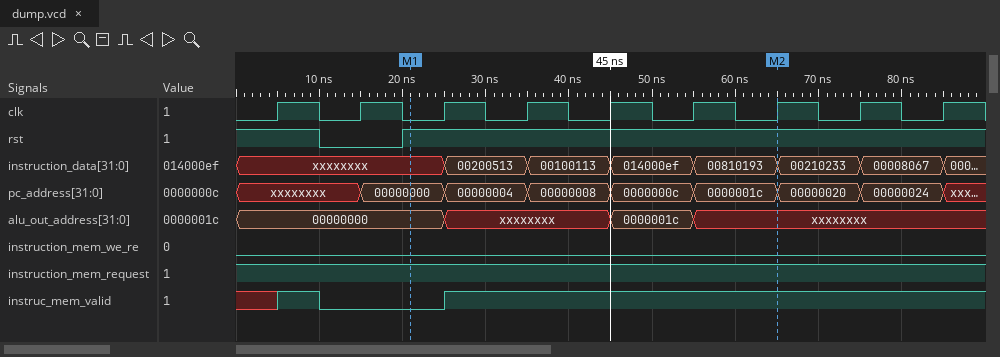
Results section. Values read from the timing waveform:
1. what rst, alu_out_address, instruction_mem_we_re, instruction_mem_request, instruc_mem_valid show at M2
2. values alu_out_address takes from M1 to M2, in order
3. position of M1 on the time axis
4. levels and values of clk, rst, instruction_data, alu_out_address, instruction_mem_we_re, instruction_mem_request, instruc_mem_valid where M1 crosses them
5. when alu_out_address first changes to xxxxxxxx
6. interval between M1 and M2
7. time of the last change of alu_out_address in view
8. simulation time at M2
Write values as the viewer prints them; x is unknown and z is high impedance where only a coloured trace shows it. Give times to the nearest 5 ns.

rst=1, alu_out_address=xxxxxxxx, instruction_mem_we_re=0, instruction_mem_request=1, instruc_mem_valid=1
00000000, xxxxxxxx, 0000001c, xxxxxxxx
20 ns
clk=0, rst=1, instruction_data=xxxxxxxx, alu_out_address=00000000, instruction_mem_we_re=0, instruction_mem_request=1, instruc_mem_valid=0
25 ns
45 ns
55 ns
65 ns
